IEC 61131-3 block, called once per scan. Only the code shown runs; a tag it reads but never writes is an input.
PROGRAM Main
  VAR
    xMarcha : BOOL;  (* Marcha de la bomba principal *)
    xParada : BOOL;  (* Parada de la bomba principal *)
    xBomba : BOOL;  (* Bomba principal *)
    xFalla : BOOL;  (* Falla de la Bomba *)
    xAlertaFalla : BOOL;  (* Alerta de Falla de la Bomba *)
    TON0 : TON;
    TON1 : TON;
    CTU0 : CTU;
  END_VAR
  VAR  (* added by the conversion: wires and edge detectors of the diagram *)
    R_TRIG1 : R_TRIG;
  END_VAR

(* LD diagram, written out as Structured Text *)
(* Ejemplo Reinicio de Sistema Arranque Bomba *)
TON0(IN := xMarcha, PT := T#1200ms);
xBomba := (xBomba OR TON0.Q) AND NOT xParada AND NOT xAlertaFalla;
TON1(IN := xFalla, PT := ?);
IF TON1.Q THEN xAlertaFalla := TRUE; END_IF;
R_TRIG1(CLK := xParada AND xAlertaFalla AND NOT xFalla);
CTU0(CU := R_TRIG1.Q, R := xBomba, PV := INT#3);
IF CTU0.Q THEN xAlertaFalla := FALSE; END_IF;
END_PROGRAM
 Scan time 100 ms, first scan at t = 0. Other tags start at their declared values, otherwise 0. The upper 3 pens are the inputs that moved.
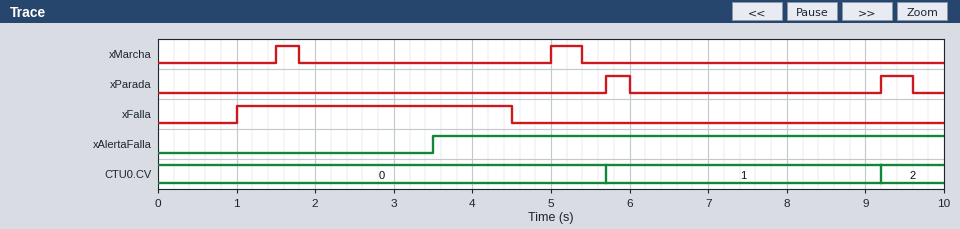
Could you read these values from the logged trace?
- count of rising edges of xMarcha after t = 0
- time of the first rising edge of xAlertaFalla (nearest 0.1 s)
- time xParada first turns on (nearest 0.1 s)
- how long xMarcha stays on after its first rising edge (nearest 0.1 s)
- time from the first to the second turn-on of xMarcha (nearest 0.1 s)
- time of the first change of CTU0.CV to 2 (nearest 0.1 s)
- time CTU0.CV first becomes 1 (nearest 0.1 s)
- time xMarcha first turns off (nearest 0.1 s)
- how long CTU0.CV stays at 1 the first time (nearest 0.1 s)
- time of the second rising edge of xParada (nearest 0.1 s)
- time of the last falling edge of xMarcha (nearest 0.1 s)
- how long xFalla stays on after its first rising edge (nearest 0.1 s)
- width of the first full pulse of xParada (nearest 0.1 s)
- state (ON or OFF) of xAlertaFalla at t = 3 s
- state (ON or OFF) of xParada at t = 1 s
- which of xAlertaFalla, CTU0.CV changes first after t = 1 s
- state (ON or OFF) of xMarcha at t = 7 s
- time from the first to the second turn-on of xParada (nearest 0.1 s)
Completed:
2
3.5 s
5.7 s
0.3 s
3.5 s
9.2 s
5.7 s
1.8 s
3.5 s
9.2 s
5.4 s
3.5 s
0.3 s
OFF
OFF
xAlertaFalla
OFF
3.5 s
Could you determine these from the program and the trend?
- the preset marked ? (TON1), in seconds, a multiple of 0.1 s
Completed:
2.5 s
